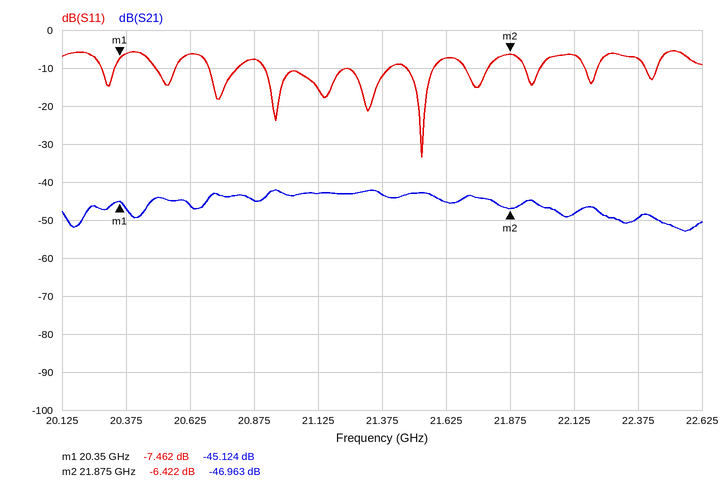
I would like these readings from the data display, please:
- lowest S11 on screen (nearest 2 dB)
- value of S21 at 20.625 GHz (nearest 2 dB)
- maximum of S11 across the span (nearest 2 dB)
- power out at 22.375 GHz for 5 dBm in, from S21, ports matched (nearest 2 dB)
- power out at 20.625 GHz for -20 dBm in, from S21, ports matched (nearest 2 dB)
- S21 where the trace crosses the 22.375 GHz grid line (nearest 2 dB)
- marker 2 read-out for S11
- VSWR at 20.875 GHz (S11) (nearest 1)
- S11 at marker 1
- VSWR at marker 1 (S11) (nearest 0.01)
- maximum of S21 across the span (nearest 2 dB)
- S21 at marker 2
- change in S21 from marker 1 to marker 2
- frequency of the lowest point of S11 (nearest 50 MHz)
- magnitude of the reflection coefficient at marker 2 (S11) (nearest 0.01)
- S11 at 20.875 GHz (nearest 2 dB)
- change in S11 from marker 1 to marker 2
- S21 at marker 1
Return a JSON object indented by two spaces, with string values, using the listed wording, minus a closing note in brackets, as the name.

{
  "lowest S11 on screen": "-34 dB",
  "value of S21 at 20.625 GHz": "-46 dB",
  "maximum of S11 across the span": "-6 dB",
  "power out at 22.375 GHz for 5 dBm in, from S21, ports matched": "-44 dBm",
  "power out at 20.625 GHz for -20 dBm in, from S21, ports matched": "-66 dBm",
  "S21 where the trace crosses the 22.375 GHz grid line": "-50 dB",
  "marker 2 read-out for S11": "-6.422 dB",
  "VSWR at 20.875 GHz (S11)": "2",
  "S11 at marker 1": "-7.462 dB",
  "VSWR at marker 1 (S11)": "2.47",
  "maximum of S21 across the span": "-42 dB",
  "S21 at marker 2": "-46.963 dB",
  "change in S21 from marker 1 to marker 2": "-1.839 dB",
  "frequency of the lowest point of S11": "21.55 GHz",
  "magnitude of the reflection coefficient at marker 2 (S11)": "0.48",
  "S11 at 20.875 GHz": "-8 dB",
  "change in S11 from marker 1 to marker 2": "1.040 dB",
  "S21 at marker 1": "-45.124 dB"
}
